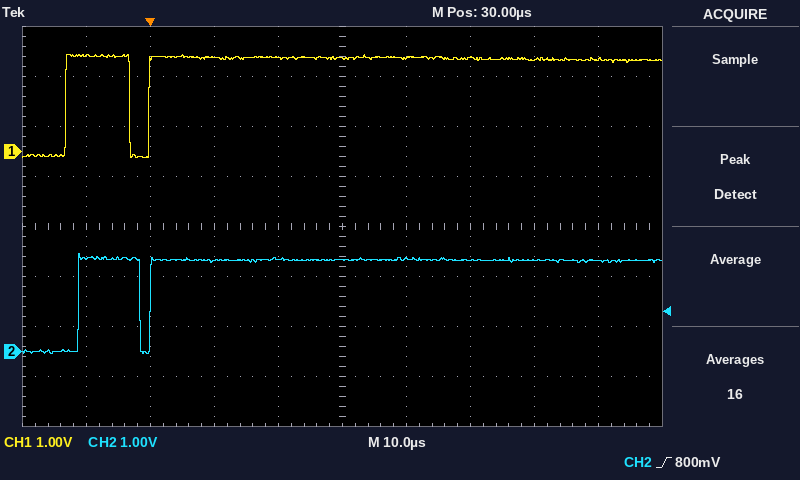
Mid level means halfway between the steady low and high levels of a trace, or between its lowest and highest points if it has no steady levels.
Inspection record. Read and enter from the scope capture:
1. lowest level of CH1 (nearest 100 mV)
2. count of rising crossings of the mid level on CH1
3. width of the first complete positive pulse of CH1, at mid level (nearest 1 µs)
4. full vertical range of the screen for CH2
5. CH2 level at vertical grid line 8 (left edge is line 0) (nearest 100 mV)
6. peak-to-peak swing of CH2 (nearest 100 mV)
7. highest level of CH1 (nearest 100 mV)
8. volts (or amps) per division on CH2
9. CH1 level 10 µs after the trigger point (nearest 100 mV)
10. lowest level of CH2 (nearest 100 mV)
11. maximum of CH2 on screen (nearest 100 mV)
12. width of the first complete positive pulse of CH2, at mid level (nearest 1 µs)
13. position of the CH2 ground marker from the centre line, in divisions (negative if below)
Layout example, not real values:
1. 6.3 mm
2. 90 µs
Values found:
1. -100 mV
2. 2
3. 10 µs
4. 8 V
5. 1.8 V
6. 2.0 V
7. 1.9 V
8. 1 V
9. 1.9 V
10. 0.0 V
11. 2.0 V
12. 10 µs
13. -2.5 div
